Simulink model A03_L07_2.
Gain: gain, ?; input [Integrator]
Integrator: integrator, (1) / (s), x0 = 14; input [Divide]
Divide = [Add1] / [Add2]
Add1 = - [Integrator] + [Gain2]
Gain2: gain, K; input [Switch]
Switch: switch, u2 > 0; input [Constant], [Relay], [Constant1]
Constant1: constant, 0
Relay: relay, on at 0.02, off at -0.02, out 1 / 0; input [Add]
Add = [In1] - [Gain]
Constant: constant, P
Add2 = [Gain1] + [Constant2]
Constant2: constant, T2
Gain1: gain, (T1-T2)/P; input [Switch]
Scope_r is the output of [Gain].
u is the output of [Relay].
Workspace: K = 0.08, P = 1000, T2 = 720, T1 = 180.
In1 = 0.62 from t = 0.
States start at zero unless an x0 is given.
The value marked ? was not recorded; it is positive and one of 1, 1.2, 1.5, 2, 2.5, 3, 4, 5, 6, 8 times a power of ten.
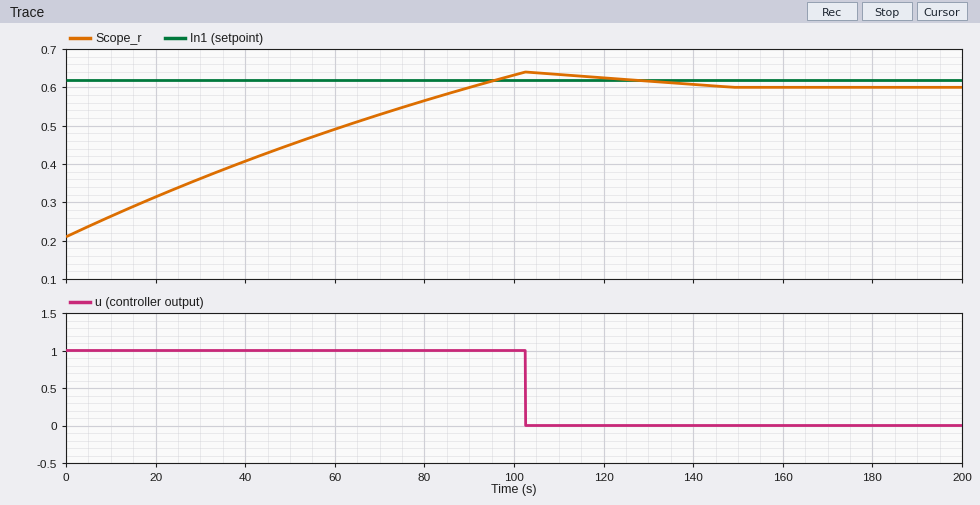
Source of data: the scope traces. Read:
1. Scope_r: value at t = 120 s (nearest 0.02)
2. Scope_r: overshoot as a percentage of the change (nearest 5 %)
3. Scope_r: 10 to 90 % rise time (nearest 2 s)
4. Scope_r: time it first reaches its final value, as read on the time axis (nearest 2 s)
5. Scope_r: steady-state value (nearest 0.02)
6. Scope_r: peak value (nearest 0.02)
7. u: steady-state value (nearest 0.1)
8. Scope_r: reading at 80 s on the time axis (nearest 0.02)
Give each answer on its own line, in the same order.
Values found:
0.62
10 %
72 s
90 s
0.60
0.64
0.0
0.56
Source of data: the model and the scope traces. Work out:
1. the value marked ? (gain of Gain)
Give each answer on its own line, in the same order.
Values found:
0.015
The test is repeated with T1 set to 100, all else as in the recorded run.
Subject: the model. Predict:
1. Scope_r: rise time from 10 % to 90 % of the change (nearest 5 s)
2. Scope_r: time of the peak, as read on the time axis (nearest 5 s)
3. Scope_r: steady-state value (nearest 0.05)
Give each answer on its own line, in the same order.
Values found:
40 s
55 s
0.60
